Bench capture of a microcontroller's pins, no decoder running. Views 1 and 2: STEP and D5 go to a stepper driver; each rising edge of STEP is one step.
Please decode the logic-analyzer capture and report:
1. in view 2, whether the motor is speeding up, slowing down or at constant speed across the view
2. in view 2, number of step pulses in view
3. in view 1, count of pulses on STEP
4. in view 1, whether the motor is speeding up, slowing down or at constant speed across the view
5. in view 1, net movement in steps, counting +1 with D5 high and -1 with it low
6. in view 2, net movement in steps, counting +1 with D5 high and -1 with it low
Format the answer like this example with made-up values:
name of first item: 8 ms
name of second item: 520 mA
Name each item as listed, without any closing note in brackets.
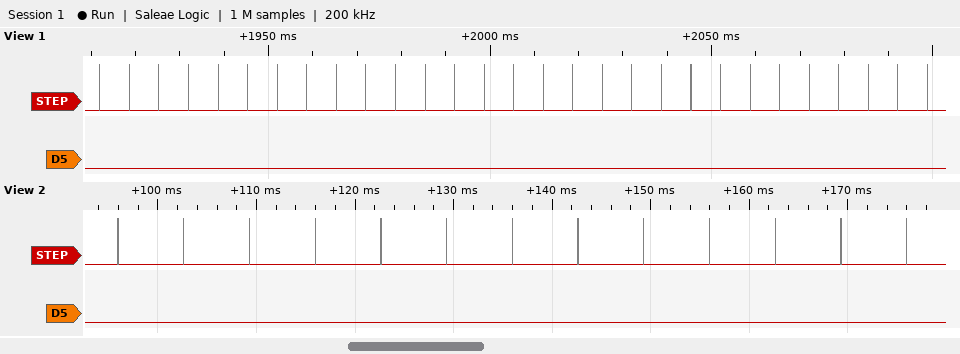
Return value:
in view 2, whether the motor is speeding up, slowing down or at constant speed across the view: constant speed
in view 2, number of step pulses in view: 13
in view 1, count of pulses on STEP: 29
in view 1, whether the motor is speeding up, slowing down or at constant speed across the view: constant speed
in view 1, net movement in steps, counting +1 with D5 high and -1 with it low: -29
in view 2, net movement in steps, counting +1 with D5 high and -1 with it low: -13
